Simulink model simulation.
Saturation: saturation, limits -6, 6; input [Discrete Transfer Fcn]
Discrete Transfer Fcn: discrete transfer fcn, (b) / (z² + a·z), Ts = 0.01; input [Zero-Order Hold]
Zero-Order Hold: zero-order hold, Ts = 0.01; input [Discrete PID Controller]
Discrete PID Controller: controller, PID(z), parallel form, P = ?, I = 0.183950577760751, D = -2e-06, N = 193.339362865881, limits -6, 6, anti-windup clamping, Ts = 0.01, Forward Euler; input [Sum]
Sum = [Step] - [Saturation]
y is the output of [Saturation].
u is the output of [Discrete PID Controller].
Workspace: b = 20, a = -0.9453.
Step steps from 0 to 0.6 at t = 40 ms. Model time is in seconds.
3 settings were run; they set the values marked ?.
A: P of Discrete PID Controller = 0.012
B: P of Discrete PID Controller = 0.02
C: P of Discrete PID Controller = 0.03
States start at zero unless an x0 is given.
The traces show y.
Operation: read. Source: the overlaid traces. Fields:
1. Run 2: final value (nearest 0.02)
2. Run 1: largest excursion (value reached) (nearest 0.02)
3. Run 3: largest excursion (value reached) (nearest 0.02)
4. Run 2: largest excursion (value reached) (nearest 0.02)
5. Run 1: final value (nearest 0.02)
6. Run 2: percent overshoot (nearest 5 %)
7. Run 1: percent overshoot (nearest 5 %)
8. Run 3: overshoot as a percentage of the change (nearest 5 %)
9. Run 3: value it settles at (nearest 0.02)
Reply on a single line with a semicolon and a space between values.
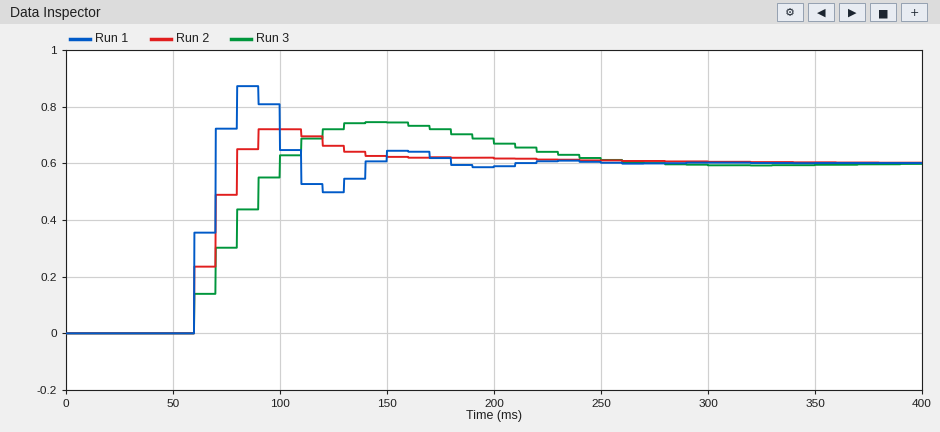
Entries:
0.60; 0.88; 0.74; 0.72; 0.60; 20 %; 45 %; 25 %; 0.60
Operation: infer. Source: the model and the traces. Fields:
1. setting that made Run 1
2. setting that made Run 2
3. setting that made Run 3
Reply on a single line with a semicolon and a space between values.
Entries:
C; B; A
